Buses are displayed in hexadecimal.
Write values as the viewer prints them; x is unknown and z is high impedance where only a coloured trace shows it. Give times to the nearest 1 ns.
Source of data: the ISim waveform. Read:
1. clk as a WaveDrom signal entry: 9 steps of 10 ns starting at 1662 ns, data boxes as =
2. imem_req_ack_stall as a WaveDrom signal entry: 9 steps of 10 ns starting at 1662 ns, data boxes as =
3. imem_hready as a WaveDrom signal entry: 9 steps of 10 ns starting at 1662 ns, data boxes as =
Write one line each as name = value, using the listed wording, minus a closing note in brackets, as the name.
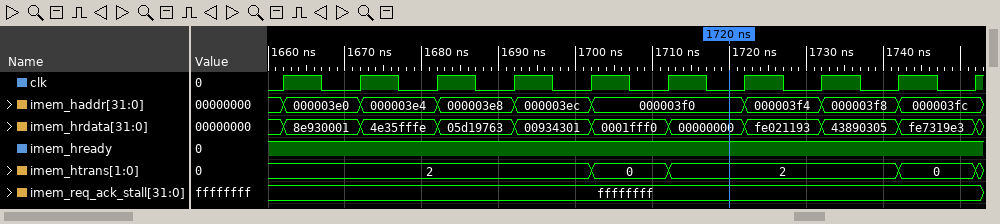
clk as a WaveDrom signal entry: 9 steps of 10 ns starting at 1662 ns, data boxes as = = {name: 'clk', wave: 'p........'}
imem_req_ack_stall as a WaveDrom signal entry: 9 steps of 10 ns starting at 1662 ns, data boxes as = = {name: 'imem_req_ack_stall', wave: '=........', data: 'ffffffff'}
imem_hready as a WaveDrom signal entry: 9 steps of 10 ns starting at 1662 ns, data boxes as = = {name: 'imem_hready', wave: '1........'}
